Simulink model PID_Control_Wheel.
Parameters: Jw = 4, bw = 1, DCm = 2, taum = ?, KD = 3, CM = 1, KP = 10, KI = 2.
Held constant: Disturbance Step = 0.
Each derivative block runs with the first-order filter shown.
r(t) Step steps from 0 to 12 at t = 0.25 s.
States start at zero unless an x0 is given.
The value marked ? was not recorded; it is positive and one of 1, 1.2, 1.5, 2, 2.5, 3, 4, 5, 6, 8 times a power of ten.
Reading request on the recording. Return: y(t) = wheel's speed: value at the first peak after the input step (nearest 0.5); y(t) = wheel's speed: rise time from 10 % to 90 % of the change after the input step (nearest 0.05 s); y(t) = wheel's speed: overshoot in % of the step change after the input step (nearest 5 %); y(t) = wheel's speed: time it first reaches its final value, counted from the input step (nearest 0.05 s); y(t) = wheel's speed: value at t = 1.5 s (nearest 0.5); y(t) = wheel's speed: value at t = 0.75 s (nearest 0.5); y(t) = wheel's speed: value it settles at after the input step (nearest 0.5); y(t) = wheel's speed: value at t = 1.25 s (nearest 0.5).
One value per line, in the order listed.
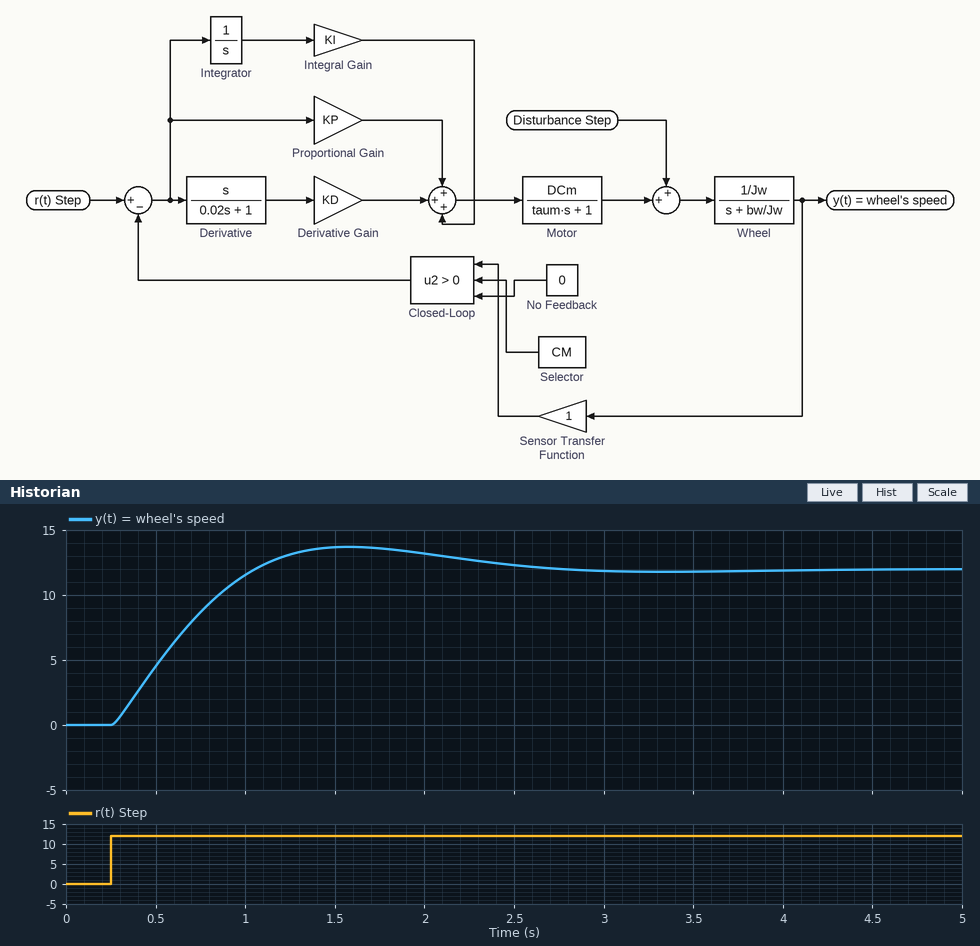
13.5
0.60 s
15 %
0.80 s
13.5
8.5
12.0
13.0
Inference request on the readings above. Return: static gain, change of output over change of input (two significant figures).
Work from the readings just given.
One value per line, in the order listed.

1.0
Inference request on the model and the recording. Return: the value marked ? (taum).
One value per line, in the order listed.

1
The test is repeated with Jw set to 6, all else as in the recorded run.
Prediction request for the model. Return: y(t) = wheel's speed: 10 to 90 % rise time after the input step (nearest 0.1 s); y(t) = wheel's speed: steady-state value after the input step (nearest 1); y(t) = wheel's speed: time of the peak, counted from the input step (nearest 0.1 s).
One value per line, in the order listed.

0.8 s
12
1.7 s
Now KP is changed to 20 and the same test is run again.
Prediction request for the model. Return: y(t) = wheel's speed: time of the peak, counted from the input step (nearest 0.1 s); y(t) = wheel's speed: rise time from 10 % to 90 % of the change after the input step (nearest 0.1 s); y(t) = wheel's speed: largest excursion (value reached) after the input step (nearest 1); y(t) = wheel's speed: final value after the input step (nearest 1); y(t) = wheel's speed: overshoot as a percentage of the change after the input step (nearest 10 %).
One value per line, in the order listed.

0.9 s
0.4 s
15
12
30 %
